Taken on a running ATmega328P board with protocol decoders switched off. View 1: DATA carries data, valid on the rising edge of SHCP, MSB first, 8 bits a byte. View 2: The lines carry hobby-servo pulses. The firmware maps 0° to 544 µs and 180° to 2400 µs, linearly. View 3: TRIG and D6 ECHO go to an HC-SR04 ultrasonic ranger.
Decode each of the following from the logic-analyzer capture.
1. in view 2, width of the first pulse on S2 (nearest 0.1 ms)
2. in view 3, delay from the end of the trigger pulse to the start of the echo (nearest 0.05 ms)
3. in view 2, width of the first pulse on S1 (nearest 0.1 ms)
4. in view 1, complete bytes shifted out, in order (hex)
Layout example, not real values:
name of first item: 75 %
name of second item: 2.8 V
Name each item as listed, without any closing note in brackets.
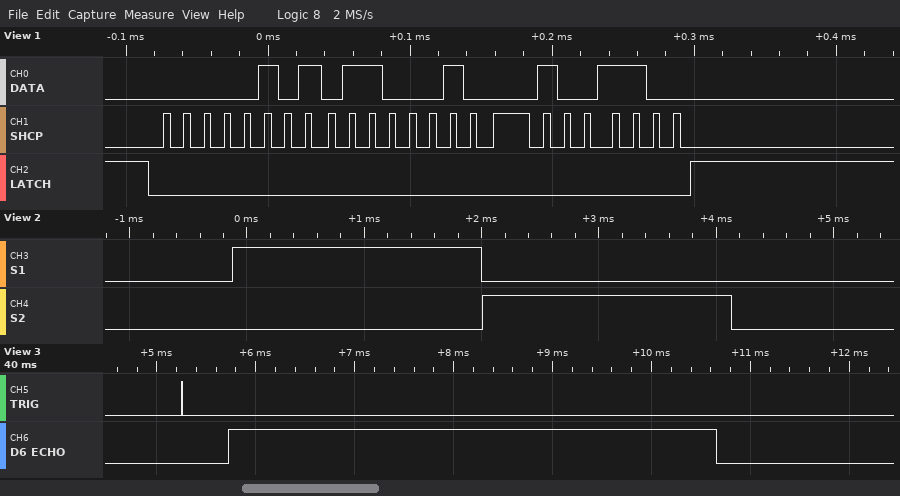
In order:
in view 2, width of the first pulse on S2: 2.1 ms
in view 3, delay from the end of the trigger pulse to the start of the echo: 0.45 ms
in view 2, width of the first pulse on S1: 2.1 ms
in view 1, complete bytes shifted out, in order: 0x05 0x62 0x4C
